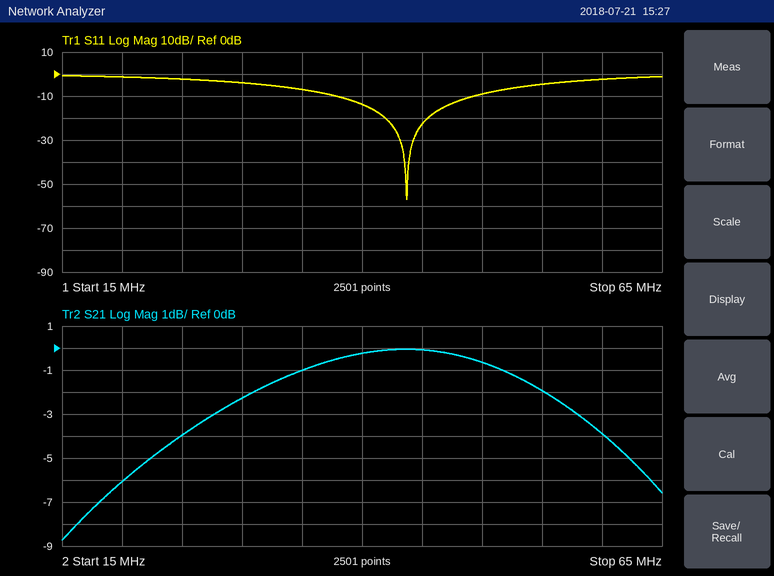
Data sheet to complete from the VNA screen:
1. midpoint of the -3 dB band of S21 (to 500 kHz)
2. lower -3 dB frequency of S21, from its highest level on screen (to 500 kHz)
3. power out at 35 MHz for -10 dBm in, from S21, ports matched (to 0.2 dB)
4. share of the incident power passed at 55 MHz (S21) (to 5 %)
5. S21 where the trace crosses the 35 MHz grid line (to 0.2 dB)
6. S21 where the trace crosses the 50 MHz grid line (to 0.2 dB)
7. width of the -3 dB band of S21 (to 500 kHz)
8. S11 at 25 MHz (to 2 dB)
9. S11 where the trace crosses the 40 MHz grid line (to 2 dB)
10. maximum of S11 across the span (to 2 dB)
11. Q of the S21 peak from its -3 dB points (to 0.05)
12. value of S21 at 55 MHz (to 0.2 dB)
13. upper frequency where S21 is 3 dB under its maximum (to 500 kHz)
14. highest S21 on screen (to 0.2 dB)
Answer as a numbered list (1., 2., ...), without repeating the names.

1. 43.0 MHz
2. 27.5 MHz
3. -11.0 dBm
4. 65 %
5. -1.0 dB
6. -0.6 dB
7. 30.5 MHz
8. -2 dB
9. -14 dB
10. 0 dB
11. 1.40
12. -2.0 dB
13. 58.0 MHz
14. 0.0 dB
